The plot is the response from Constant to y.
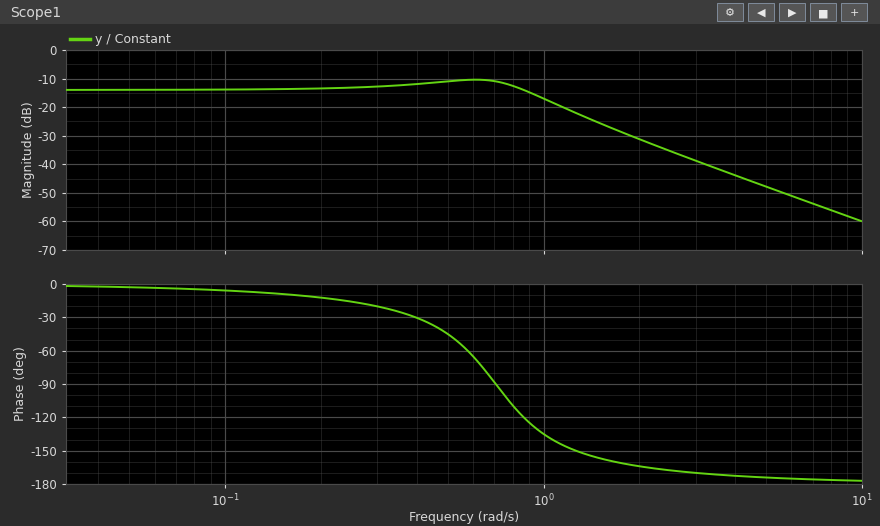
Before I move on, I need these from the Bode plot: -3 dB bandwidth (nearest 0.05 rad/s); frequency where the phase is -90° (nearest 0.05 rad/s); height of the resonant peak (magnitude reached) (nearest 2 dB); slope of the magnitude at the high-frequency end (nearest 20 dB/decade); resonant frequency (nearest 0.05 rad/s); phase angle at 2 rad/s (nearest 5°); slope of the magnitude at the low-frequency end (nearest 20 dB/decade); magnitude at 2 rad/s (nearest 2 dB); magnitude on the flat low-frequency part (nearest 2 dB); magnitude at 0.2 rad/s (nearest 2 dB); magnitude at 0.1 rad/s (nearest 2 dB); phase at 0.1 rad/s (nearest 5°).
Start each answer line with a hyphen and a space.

- 1.00 rad/s
- 0.70 rad/s
- -10 dB
- -40 dB/decade
- 0.60 rad/s
- -165°
- 0 dB/decade
- -32 dB
- -14 dB
- -14 dB
- -14 dB
- -5°
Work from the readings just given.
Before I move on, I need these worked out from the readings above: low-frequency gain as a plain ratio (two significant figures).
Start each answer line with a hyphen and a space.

- 0.20
